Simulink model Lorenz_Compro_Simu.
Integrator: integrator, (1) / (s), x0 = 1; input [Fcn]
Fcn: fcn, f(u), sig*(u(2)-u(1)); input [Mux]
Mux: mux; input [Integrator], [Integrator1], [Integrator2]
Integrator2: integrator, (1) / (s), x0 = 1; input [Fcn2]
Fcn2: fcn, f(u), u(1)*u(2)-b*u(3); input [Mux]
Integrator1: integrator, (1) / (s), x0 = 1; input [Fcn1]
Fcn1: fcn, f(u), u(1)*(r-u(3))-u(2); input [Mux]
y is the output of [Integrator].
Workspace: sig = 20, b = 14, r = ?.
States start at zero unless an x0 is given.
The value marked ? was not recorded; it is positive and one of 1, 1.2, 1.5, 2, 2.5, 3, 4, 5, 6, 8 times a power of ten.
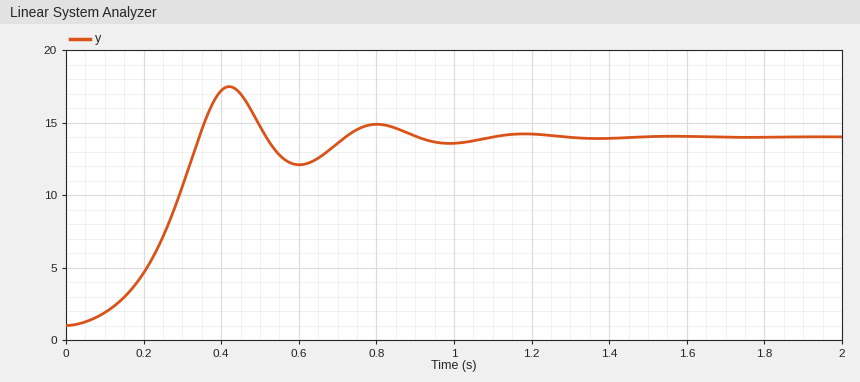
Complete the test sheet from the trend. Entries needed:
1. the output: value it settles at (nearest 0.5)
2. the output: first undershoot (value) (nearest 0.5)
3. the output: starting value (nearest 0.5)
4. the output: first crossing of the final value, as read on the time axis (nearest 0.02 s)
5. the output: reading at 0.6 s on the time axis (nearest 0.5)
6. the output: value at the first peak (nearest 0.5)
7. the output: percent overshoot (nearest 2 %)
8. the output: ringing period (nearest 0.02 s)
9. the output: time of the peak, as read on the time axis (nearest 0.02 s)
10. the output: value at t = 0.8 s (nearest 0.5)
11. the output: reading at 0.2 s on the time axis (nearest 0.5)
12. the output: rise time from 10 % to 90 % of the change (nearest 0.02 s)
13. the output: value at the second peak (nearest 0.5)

14.0
12.0
1.0
0.34 s
12.0
17.5
26 %
0.38 s
0.42 s
15.0
4.5
0.20 s
15.0
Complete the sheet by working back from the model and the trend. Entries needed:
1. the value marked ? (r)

15
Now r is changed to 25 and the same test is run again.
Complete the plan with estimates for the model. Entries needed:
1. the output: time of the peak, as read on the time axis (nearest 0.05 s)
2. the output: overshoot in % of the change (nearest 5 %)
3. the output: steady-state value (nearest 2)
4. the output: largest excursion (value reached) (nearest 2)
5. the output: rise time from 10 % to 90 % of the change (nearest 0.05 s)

0.30 s
40 %
18
26
0.15 s
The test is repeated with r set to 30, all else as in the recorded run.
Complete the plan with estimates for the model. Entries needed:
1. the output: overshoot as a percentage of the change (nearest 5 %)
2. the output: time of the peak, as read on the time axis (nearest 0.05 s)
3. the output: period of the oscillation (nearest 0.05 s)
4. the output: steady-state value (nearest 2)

45 %
0.30 s
0.30 s
20
